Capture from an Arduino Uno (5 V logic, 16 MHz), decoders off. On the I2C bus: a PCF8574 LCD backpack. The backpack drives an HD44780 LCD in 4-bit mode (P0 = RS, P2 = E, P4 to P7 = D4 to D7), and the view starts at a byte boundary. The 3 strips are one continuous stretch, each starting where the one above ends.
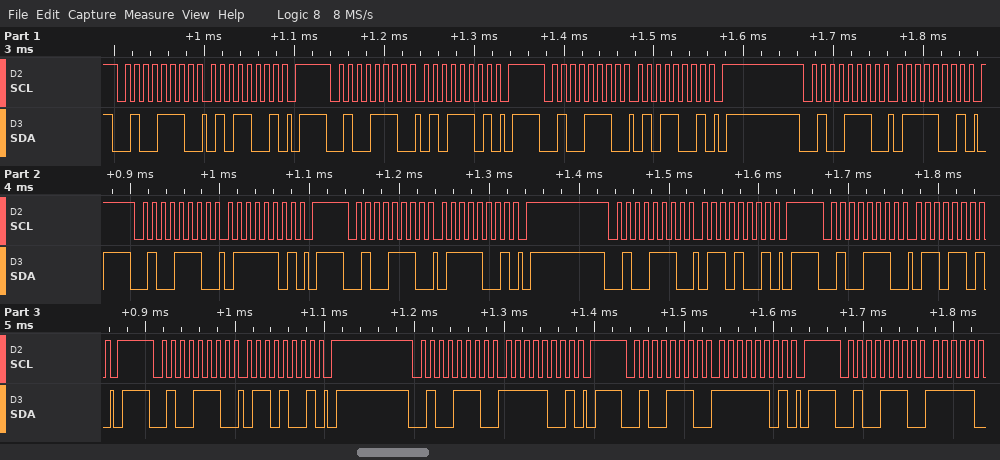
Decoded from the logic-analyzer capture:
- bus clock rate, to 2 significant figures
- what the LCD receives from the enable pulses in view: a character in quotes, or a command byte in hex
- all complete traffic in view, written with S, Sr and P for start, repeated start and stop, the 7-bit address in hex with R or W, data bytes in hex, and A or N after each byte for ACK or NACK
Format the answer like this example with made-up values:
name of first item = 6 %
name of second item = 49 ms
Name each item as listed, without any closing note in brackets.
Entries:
bus clock rate, to 2 significant figures = 100 kHz
what the LCD receives from the enable pulses in view: a character in quotes, or a command byte in hex = 'W'
all complete traffic in view, written with S, Sr and P for start, repeated start and stop, the 7-bit address in hex with R or W, data bytes in hex, and A or N after each byte for ACK or NACK = S 27W A 59 A P S 27W A 5D A P S 27W A 59 A P S 27W A 79 A P S 27W A 7D A P S 27W A 79 A P S 27W A 69 A P S 27W A 6D A P S 27W A 69 A P S 27W A F9 A P S 27W A FD A P S 27W A
